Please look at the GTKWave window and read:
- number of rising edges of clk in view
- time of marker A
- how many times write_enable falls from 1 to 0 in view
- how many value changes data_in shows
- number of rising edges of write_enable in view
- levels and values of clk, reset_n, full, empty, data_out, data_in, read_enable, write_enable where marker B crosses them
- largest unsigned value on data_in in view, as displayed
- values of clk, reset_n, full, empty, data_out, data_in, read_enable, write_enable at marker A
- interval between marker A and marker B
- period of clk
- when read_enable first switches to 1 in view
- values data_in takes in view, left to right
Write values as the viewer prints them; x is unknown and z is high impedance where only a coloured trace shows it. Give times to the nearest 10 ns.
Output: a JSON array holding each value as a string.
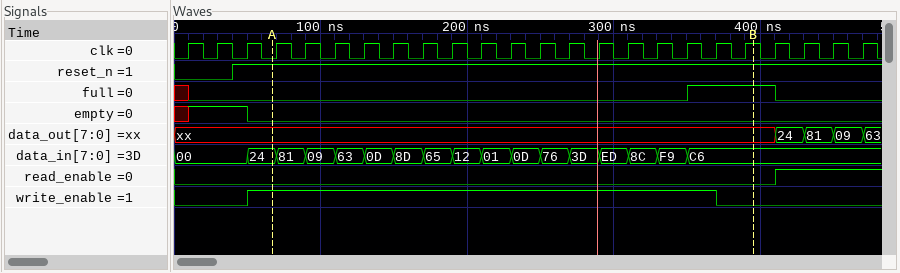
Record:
["24", "70 ns", "1", "16", "1", "clk=1, reset_n=1, full=1, empty=0, data_out=xx, data_in=C6, read_enable=0, write_enable=0", "F9", "clk=0, reset_n=1, full=0, empty=0, data_out=xx, data_in=24, read_enable=0, write_enable=1", "330 ns", "20 ns", "410 ns", "00, 24, 81, 09, 63, 0D, 8D, 65, 12, 01, 0D, 76, 3D, ED, 8C, F9, C6"]
